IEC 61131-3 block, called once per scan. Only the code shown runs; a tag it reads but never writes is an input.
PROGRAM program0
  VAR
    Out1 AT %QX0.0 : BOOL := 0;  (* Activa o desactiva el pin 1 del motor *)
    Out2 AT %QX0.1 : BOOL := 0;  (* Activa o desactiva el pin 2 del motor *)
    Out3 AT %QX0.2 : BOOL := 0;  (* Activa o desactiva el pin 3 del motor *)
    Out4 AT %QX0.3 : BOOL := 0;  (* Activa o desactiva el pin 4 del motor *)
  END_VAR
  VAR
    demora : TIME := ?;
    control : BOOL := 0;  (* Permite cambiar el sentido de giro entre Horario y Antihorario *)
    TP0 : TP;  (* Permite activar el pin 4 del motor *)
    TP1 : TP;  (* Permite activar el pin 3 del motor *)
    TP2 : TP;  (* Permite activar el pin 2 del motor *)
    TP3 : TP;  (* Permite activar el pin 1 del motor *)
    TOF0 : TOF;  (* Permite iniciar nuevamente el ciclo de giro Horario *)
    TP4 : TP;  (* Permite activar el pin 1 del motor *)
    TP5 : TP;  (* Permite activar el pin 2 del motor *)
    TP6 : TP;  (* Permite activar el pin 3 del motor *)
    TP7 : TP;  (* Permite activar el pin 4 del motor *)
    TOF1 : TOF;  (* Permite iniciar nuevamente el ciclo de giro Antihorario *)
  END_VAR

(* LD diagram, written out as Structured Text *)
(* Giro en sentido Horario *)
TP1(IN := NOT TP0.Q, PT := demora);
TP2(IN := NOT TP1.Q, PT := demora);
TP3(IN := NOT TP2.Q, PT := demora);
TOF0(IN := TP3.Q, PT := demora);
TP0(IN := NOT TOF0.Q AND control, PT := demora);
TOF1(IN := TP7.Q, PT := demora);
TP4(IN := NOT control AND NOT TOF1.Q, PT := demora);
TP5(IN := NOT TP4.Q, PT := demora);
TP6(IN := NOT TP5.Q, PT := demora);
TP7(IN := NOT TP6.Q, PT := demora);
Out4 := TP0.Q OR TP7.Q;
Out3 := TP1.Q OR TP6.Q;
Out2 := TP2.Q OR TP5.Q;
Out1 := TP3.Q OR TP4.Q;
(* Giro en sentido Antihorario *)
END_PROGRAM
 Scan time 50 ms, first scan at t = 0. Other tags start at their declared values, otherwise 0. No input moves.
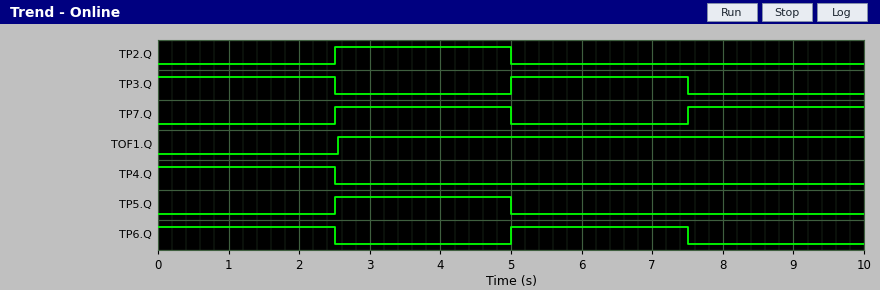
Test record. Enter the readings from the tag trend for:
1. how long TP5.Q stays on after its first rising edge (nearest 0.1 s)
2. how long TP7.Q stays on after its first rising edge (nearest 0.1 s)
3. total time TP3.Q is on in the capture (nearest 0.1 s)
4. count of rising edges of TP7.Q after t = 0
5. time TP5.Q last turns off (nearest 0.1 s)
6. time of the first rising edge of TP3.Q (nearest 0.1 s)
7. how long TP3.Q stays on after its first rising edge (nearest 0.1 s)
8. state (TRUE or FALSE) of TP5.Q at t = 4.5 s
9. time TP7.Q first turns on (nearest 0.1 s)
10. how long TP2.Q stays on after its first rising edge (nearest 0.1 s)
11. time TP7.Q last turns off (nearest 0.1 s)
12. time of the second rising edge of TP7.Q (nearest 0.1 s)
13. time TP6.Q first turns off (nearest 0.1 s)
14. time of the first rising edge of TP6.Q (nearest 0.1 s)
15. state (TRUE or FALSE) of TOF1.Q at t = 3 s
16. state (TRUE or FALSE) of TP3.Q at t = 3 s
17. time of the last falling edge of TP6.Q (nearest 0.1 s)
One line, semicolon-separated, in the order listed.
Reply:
2.5 s; 2.5 s; 5.0 s; 2; 5.0 s; 5.0 s; 2.5 s; TRUE; 2.5 s; 2.5 s; 5.0 s; 7.5 s; 2.5 s; 5.0 s; TRUE; FALSE; 7.5 s
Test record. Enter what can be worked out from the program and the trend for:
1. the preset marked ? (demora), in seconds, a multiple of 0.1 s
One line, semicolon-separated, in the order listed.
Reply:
2.5 s
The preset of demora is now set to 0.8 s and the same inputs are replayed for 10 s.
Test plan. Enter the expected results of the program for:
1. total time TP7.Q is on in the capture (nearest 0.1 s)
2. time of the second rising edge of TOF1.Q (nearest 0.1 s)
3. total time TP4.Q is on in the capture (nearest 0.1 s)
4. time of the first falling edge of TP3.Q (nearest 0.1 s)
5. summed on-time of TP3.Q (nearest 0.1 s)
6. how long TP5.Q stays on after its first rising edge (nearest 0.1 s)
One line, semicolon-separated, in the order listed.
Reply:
2.4 s; 6.5 s; 2.4 s; 0.8 s; 1.6 s; 0.8 s
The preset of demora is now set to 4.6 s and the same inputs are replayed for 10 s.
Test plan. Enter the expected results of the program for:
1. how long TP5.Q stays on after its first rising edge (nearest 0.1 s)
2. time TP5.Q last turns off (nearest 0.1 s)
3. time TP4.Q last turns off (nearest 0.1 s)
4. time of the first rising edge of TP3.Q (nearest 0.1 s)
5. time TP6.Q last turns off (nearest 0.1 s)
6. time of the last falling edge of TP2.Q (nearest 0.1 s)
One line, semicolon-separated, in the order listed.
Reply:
4.6 s; 9.2 s; 4.6 s; 9.2 s; 4.6 s; 9.2 s
